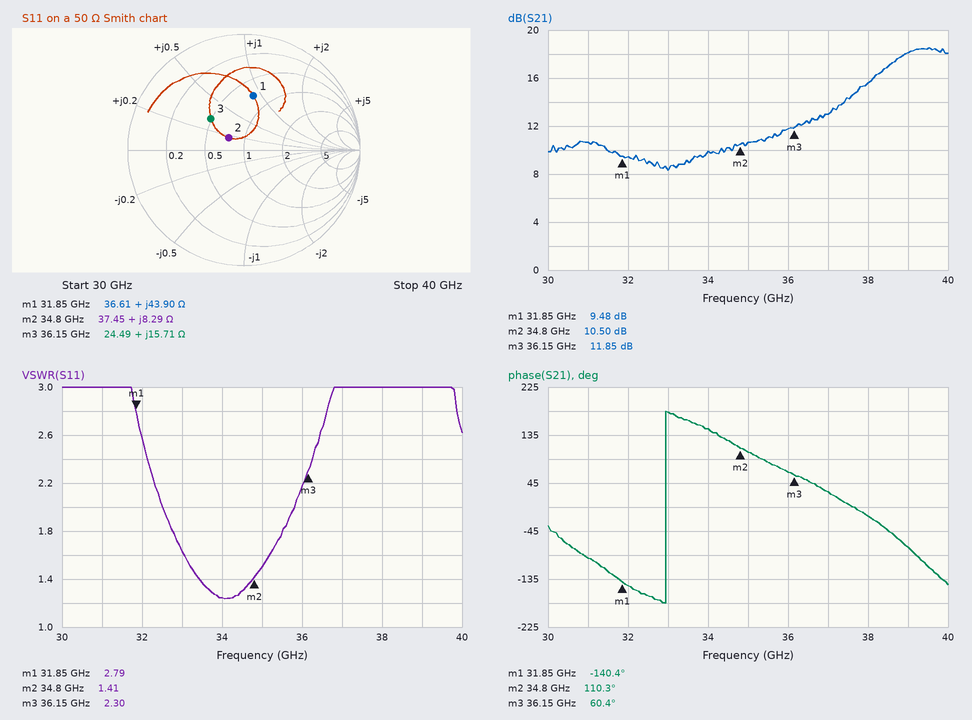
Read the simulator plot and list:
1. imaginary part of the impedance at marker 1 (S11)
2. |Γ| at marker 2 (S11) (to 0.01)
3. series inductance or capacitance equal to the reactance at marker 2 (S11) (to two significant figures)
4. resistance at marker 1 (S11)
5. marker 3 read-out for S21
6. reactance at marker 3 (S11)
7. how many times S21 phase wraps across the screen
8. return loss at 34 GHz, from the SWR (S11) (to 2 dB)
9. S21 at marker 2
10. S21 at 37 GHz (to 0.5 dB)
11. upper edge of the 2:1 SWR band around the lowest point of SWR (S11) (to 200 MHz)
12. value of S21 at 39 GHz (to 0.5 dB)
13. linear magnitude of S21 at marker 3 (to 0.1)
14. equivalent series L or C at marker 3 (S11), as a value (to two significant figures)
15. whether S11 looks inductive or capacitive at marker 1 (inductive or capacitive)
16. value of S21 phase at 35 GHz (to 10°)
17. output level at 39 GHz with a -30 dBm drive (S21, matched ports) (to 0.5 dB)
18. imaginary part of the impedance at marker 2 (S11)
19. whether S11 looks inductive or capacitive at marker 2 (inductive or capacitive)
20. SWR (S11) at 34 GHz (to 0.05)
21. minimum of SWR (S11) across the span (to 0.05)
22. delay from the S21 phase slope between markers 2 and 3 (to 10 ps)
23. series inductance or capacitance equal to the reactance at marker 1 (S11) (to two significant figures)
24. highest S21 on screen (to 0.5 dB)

+43.90 Ω
0.17
38 pH
36.61 Ω
11.85 dB
+15.71 Ω
1
20 dB
10.50 dB
13.0 dB
35.8 GHz
18.0 dB
3.9
69 pH
inductive
100°
-12.0 dBm
+8.29 Ω
inductive
1.25
1.25
100 ps
220 pH
18.5 dB
